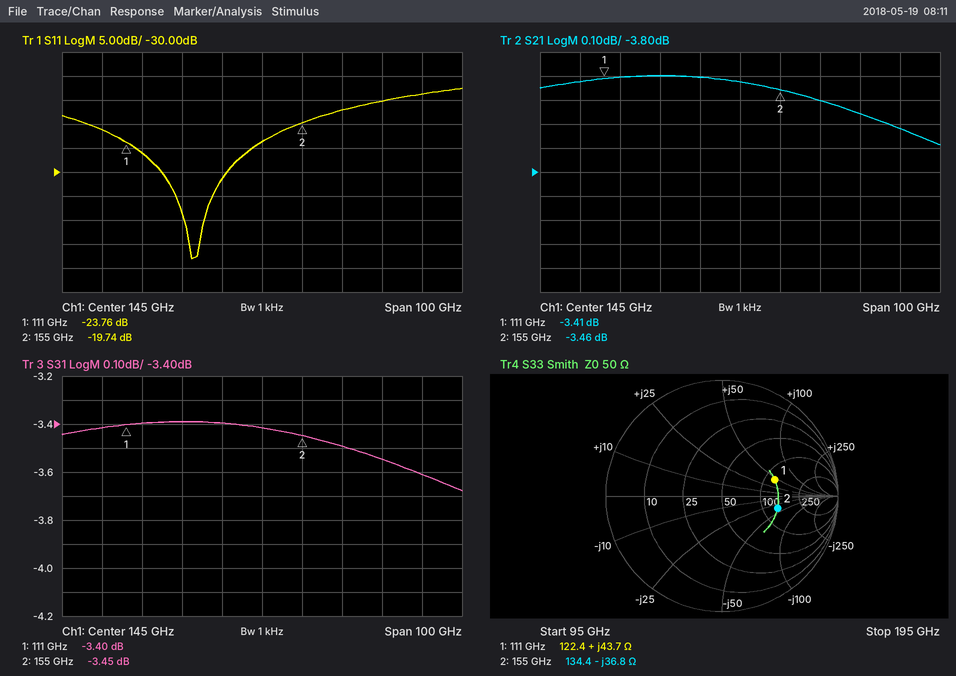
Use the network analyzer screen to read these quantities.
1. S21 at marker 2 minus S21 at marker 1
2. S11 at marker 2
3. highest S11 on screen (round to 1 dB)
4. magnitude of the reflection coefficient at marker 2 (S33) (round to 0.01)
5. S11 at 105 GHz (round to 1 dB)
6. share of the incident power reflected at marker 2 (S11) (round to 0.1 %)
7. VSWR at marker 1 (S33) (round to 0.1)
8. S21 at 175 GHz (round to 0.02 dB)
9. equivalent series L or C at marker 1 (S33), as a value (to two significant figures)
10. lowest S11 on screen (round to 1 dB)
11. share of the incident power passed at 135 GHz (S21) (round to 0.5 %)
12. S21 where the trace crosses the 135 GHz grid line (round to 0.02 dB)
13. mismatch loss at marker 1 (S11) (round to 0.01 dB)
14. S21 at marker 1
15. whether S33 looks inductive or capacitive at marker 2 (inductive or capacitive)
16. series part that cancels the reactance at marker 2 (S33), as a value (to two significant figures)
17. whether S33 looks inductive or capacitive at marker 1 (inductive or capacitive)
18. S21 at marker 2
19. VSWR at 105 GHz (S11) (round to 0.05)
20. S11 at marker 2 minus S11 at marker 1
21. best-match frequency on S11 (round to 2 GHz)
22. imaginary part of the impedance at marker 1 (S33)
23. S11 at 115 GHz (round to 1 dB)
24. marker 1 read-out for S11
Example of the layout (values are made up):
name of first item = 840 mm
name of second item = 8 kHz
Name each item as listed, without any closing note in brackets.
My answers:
S21 at marker 2 minus S21 at marker 1 = -0.05 dB
S11 at marker 2 = -19.74 dB
highest S11 on screen = -13 dB
magnitude of the reflection coefficient at marker 2 (S33) = 0.49
S11 at 105 GHz = -21 dB
share of the incident power reflected at marker 2 (S11) = 1.1 %
VSWR at marker 1 (S33) = 2.8
S21 at 175 GHz = -3.56 dB
equivalent series L or C at marker 1 (S33), as a value = 63 pH
lowest S11 on screen = -48 dB
share of the incident power passed at 135 GHz (S21) = 45.5 %
S21 where the trace crosses the 135 GHz grid line = -3.40 dB
mismatch loss at marker 1 (S11) = 0.02 dB
S21 at marker 1 = -3.41 dB
whether S33 looks inductive or capacitive at marker 2 = capacitive
series part that cancels the reactance at marker 2 (S33), as a value = 38 pH
whether S33 looks inductive or capacitive at marker 1 = inductive
S21 at marker 2 = -3.46 dB
VSWR at 105 GHz (S11) = 1.20
S11 at marker 2 minus S11 at marker 1 = 4.02 dB
best-match frequency on S11 = 128 GHz
imaginary part of the impedance at marker 1 = +43.7 Ω
S11 at 115 GHz = -26 dB
marker 1 read-out for S11 = -23.76 dB
